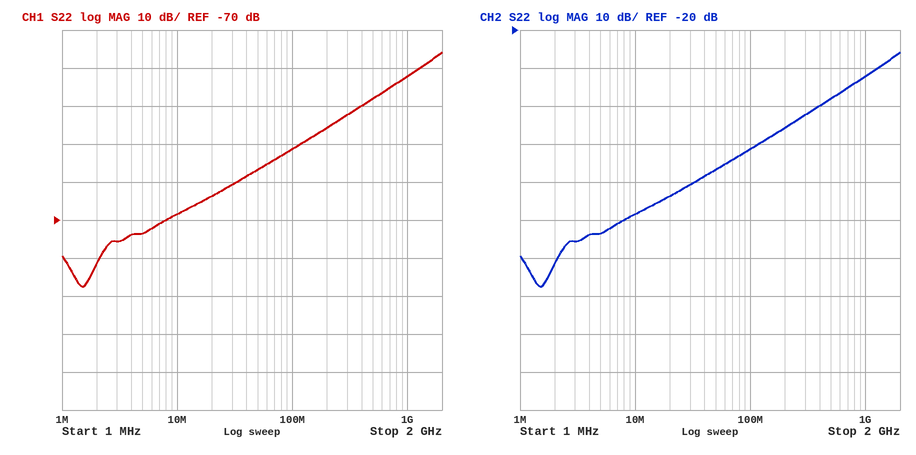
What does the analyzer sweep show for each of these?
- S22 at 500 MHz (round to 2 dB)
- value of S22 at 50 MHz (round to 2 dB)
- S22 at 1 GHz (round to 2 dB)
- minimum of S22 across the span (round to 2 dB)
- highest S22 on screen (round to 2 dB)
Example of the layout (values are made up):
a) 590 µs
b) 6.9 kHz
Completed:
a) -38 dB
b) -56 dB
c) -32 dB
d) -88 dB
e) -26 dB
